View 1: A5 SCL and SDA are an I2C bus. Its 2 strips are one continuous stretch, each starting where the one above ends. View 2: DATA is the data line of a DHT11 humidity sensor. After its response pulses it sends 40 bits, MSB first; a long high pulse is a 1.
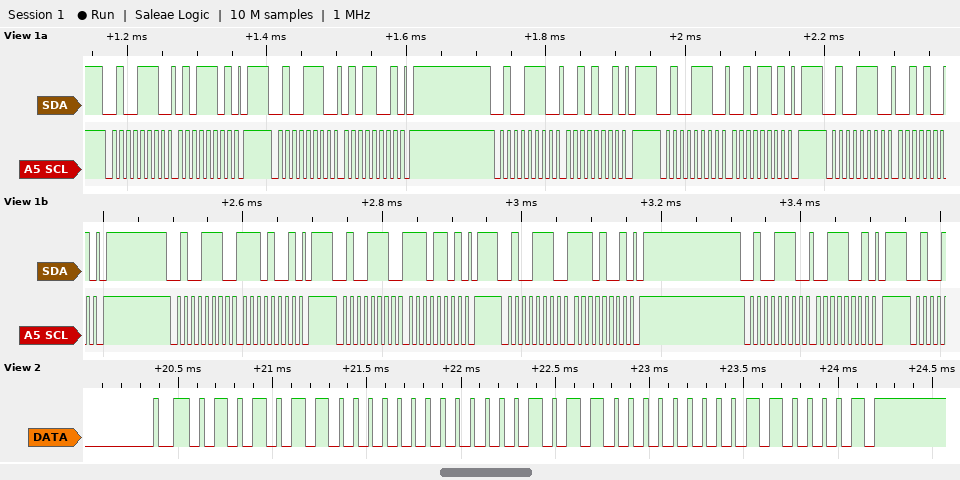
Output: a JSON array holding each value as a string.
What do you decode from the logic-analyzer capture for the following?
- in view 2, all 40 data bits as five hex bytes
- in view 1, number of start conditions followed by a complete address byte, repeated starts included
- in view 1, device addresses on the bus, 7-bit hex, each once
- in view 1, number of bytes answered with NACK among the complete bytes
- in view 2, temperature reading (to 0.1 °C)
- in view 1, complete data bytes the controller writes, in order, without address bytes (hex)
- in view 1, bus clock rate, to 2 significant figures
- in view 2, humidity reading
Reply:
["56 00 0B 00 61", "9", "0x27", "0", "11.0 °C", "5D 59 29 2D 29 E9 ED E9 39", "100 kHz", "86 %"]
